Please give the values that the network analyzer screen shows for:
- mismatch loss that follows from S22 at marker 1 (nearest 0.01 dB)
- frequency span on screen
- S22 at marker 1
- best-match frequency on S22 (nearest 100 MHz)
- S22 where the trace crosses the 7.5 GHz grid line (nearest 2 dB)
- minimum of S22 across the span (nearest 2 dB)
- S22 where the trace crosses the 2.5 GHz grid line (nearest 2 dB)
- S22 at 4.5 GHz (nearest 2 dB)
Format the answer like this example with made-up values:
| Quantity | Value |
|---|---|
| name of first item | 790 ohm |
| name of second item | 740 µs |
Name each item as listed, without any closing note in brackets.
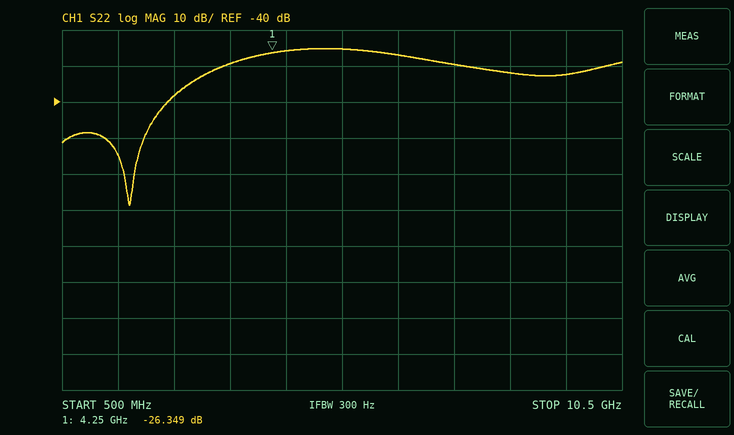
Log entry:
| Quantity | Value |
|---|---|
| mismatch loss that follows from S22 at marker 1 | 0.01 dB |
| frequency span on screen | 10 GHz |
| S22 at marker 1 | -26.349 dB |
| best-match frequency on S22 | 1.7 GHz |
| S22 where the trace crosses the 7.5 GHz grid line | -30 dB |
| minimum of S22 across the span | -68 dB |
| S22 where the trace crosses the 2.5 GHz grid line | -38 dB |
| S22 at 4.5 GHz | -26 dB |
